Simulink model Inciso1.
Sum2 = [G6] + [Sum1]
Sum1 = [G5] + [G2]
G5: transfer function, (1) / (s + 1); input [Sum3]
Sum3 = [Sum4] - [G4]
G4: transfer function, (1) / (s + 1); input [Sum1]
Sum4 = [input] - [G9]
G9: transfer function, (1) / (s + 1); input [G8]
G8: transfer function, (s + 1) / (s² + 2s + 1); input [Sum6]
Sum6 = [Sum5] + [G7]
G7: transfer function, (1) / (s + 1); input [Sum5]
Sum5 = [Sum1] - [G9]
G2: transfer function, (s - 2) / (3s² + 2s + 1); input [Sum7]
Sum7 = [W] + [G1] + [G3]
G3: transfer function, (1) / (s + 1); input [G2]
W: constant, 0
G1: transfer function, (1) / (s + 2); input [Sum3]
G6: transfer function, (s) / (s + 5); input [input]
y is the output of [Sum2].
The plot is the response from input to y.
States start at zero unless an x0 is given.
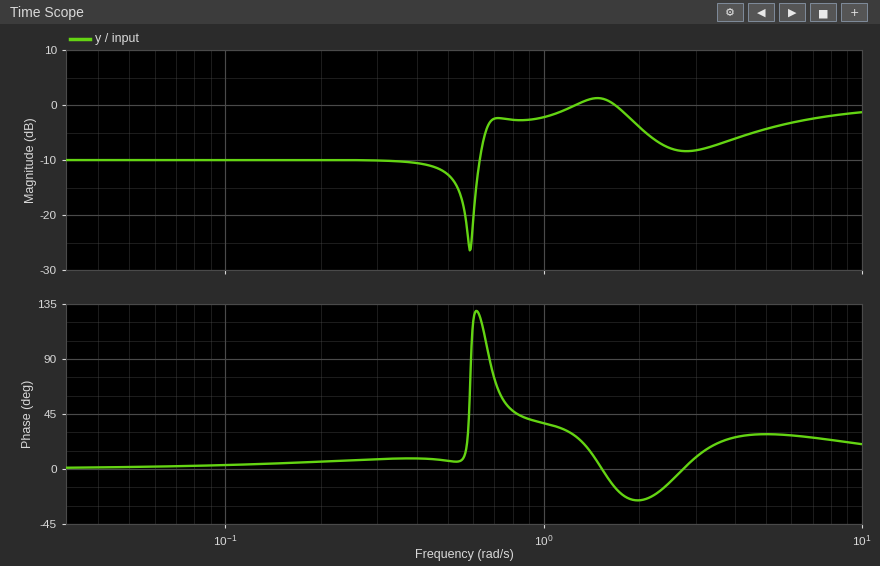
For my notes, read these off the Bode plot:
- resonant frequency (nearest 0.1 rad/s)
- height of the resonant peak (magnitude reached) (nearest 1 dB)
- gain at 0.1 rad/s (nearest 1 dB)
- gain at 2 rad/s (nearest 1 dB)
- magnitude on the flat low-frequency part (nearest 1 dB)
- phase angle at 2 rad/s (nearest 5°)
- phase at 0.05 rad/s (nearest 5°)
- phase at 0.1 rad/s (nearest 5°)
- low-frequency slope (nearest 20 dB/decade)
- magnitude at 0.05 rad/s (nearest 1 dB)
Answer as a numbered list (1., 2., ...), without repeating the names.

1. 1.5 rad/s
2. 1 dB
3. -10 dB
4. -4 dB
5. -10 dB
6. -25°
7. 0°
8. 5°
9. 0 dB/decade
10. -10 dB
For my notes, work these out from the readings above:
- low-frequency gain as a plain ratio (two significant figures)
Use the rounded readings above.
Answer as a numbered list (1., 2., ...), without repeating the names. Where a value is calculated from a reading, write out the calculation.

1. 10^(-10 / 20) = 0.32
